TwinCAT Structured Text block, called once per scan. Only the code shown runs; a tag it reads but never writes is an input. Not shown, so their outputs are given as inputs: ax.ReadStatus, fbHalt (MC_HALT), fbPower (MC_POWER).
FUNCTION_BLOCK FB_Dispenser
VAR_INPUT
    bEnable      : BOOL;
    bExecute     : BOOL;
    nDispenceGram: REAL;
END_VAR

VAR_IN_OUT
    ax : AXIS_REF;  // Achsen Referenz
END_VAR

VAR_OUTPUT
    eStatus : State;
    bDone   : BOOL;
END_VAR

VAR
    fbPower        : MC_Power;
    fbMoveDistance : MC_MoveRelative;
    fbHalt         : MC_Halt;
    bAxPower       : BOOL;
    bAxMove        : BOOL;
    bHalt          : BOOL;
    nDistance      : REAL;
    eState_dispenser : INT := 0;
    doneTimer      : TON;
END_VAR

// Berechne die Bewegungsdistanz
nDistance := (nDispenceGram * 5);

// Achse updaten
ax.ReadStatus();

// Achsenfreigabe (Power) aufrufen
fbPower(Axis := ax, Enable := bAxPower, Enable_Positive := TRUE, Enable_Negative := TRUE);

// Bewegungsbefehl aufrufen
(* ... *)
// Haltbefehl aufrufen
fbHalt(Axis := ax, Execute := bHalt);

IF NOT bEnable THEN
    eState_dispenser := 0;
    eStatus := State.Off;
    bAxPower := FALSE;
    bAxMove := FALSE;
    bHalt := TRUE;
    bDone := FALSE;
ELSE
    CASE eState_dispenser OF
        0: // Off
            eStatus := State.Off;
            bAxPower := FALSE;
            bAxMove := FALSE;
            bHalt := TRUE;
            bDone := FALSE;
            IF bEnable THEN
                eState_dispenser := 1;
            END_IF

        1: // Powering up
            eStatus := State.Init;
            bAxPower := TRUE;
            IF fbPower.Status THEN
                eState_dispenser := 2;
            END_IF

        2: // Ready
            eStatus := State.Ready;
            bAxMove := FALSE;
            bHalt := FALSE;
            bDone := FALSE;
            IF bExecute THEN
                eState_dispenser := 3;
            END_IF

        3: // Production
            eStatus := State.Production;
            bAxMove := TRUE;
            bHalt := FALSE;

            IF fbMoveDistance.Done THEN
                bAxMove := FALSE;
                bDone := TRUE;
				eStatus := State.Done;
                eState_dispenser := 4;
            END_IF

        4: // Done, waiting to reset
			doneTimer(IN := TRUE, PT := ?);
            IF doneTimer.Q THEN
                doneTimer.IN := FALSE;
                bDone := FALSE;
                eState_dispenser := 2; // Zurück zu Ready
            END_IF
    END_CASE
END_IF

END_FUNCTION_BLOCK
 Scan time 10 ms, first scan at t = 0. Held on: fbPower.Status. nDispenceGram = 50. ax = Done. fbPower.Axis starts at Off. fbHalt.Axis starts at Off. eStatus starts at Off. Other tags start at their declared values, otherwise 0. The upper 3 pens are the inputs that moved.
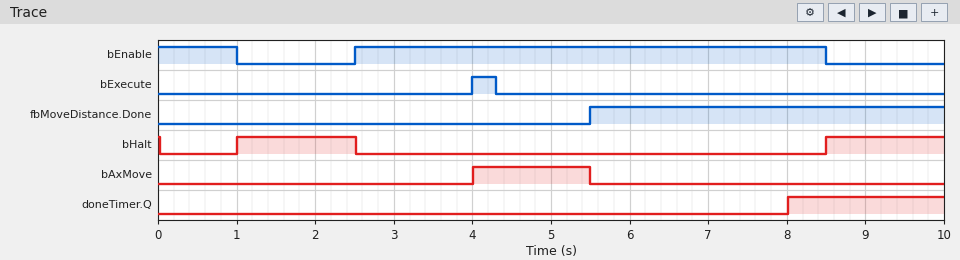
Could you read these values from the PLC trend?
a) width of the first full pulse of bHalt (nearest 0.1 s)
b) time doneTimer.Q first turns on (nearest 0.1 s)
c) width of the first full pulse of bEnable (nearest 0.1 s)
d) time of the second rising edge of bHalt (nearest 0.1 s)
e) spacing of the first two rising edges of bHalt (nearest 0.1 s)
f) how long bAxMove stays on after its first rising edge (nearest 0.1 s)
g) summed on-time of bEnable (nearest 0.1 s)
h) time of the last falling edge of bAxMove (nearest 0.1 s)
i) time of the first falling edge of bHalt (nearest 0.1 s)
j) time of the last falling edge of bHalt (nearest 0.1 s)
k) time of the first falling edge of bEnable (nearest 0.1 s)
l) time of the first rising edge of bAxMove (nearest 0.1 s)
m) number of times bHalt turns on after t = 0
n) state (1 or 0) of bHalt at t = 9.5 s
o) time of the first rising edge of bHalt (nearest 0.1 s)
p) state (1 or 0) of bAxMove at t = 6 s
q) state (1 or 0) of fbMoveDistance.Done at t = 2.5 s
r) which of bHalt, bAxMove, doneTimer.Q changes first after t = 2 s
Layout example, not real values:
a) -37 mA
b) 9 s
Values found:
a) 1.5 s
b) 8.0 s
c) 6.0 s
d) 8.5 s
e) 7.5 s
f) 1.5 s
g) 7.0 s
h) 5.5 s
i) 0.0 s
j) 2.5 s
k) 1.0 s
l) 4.0 s
m) 2
n) 1
o) 1.0 s
p) 0
q) 0
r) bHalt
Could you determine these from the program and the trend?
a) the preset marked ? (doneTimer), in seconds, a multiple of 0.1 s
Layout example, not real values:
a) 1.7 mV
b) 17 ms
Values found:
a) 2.5 s
